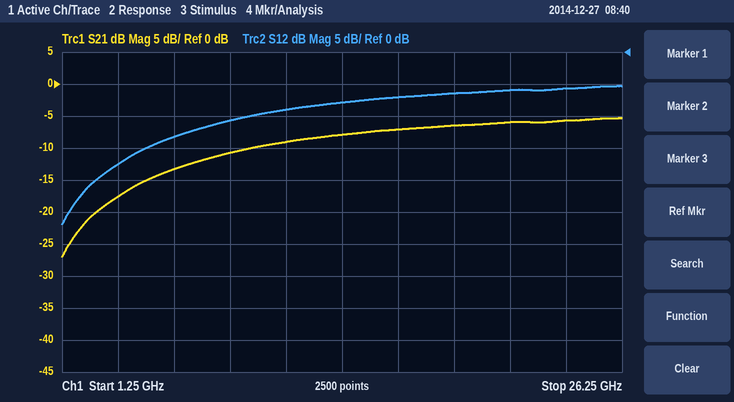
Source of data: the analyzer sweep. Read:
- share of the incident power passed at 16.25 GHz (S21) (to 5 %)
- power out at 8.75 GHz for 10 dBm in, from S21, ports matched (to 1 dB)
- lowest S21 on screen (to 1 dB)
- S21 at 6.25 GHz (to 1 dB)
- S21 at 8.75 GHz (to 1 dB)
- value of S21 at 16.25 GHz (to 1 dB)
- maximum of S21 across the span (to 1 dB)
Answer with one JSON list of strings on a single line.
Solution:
["20 %", "-1 dBm", "-27 dB", "-13 dB", "-11 dB", "-7 dB", "-5 dB"]
